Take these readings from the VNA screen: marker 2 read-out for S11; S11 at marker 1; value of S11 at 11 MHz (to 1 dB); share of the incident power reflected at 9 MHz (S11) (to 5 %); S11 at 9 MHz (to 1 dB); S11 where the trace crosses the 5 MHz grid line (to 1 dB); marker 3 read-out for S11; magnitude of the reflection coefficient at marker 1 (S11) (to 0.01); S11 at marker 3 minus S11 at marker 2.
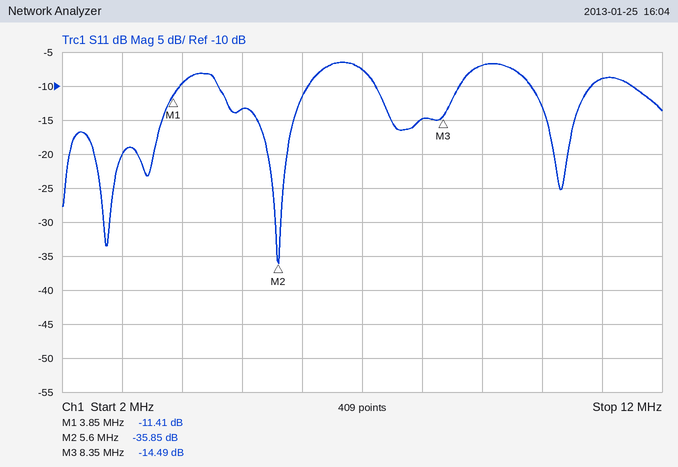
-35.85 dB
-11.41 dB
-9 dB
20 %
-7 dB
-13 dB
-14.49 dB
0.27
21.36 dB
